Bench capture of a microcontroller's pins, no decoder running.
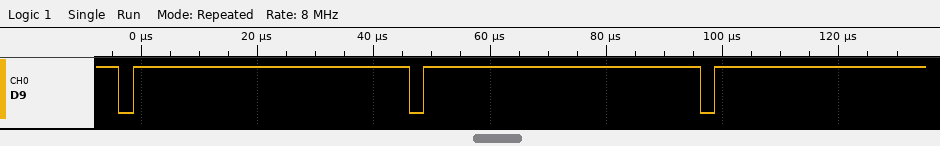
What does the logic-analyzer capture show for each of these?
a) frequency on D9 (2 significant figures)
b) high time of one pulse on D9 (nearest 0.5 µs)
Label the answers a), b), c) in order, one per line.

a) 20 kHz
b) 47.5 µs
